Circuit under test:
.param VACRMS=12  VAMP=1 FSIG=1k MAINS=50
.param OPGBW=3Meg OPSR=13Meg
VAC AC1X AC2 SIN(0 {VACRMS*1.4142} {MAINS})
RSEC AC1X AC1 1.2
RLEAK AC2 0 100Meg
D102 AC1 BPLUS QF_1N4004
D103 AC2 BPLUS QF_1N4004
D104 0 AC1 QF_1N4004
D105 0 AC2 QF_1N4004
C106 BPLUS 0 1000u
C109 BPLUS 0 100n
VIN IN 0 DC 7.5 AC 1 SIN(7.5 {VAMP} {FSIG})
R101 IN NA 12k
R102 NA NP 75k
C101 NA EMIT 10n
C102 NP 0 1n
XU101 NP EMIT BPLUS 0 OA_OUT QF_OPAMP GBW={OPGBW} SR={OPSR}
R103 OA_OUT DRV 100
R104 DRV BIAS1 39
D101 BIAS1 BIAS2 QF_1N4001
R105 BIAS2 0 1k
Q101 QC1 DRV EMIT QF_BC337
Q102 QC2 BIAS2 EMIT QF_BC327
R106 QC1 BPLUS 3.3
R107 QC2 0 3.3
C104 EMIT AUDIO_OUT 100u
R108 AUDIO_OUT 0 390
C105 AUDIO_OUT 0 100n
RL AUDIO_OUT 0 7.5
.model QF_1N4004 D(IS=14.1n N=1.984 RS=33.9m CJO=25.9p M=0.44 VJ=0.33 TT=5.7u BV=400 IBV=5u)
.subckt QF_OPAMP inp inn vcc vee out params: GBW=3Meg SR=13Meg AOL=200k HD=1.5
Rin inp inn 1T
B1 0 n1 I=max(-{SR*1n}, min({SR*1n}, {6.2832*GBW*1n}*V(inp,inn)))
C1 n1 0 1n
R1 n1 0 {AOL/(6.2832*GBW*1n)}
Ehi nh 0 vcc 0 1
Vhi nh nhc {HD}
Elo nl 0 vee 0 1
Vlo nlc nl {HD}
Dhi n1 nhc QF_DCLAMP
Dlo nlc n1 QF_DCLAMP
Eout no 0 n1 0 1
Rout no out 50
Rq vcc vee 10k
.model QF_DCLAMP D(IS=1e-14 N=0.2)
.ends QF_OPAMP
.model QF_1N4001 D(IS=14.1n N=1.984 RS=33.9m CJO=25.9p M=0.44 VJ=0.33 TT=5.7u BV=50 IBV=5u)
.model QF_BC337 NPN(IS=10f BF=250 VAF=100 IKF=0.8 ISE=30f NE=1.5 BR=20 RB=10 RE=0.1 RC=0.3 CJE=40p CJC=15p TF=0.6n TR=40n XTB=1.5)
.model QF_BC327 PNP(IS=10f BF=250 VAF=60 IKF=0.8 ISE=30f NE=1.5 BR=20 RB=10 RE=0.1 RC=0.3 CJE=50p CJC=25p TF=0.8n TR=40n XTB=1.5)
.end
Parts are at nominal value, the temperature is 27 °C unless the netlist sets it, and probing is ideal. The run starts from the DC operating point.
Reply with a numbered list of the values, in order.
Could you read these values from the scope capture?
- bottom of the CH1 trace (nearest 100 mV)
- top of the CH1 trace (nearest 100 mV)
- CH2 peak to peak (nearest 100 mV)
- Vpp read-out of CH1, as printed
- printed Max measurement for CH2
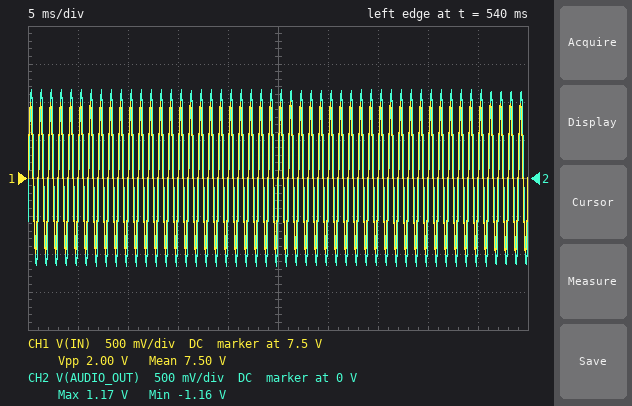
1. 6.5 V
2. 8.5 V
3. 2.3 V
4. 2.00 V
5. 1.17 V
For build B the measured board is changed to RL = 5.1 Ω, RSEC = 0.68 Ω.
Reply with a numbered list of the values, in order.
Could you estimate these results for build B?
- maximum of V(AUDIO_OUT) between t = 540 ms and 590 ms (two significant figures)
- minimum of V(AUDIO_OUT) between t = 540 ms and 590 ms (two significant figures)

1. 1.1 V
2. -1.1 V
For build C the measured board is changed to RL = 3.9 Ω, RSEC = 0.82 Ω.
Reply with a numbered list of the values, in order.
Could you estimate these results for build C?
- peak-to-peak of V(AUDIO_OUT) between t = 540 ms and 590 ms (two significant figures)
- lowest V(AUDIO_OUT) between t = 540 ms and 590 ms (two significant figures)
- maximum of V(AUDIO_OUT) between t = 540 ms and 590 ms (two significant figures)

1. 2.2 V
2. -1.1 V
3. 1.1 V
